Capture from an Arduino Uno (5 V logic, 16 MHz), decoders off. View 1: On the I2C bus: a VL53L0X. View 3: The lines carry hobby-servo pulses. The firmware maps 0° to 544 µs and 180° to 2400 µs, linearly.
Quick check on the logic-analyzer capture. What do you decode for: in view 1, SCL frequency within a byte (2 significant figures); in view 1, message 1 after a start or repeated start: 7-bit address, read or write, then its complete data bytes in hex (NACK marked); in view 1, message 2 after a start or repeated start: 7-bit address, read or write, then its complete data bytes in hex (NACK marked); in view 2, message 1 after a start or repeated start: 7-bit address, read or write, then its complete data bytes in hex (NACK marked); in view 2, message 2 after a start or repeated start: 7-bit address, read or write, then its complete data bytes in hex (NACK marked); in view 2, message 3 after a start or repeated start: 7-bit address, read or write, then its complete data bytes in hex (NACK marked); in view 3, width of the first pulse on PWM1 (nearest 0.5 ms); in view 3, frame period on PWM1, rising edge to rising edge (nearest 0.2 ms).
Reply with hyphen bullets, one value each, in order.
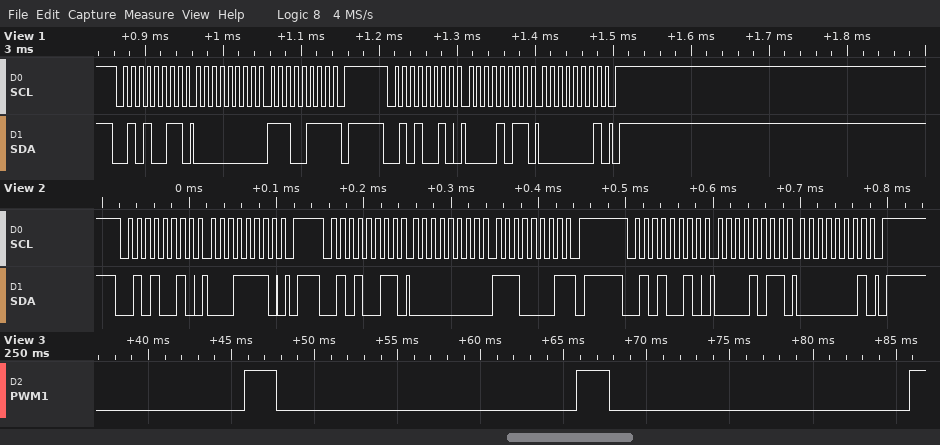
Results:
- 100 kHz
- 0x29 read: 00 E7 NACK
- 0x29 write: 0B 01
- 0x29 write: 1E
- 0x29 read: 00 E1 NACK
- 0x29 write: 0B 01
- 2.0 ms
- 20.0 ms
